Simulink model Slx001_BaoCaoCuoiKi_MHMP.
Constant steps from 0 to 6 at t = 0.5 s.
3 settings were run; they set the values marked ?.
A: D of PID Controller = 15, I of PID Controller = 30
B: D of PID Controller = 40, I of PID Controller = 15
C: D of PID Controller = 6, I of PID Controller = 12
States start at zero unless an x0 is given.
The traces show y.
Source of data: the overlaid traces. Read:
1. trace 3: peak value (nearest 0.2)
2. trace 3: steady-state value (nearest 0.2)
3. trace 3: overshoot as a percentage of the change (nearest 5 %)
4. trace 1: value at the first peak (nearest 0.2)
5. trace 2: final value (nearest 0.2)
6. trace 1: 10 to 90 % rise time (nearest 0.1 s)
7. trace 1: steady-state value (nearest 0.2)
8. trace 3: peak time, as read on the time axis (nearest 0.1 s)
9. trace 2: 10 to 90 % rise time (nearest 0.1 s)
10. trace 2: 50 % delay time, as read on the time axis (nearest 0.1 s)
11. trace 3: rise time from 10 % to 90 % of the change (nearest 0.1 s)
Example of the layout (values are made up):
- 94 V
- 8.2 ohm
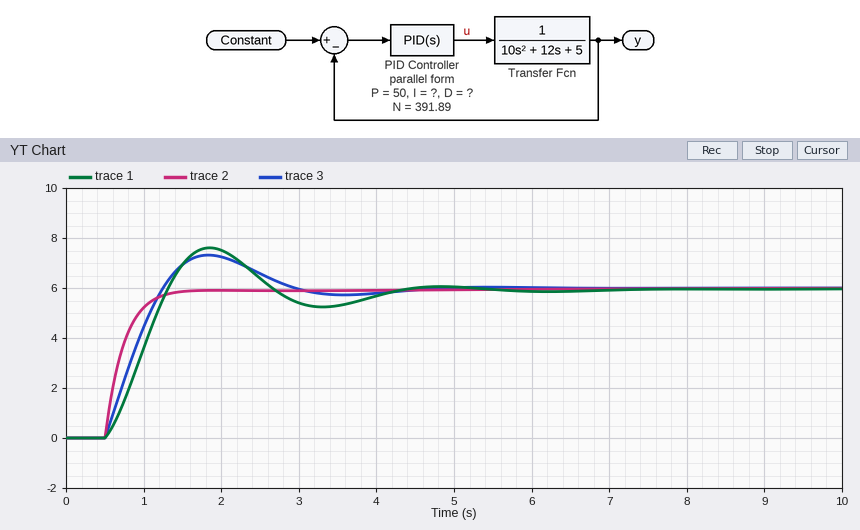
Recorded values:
- 7.4
- 6.0
- 20 %
- 7.6
- 6.0
- 0.6 s
- 6.0
- 1.8 s
- 0.5 s
- 0.7 s
- 0.6 s
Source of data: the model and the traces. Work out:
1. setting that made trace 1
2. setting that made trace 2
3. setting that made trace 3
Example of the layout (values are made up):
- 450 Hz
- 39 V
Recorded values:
- C
- B
- A
